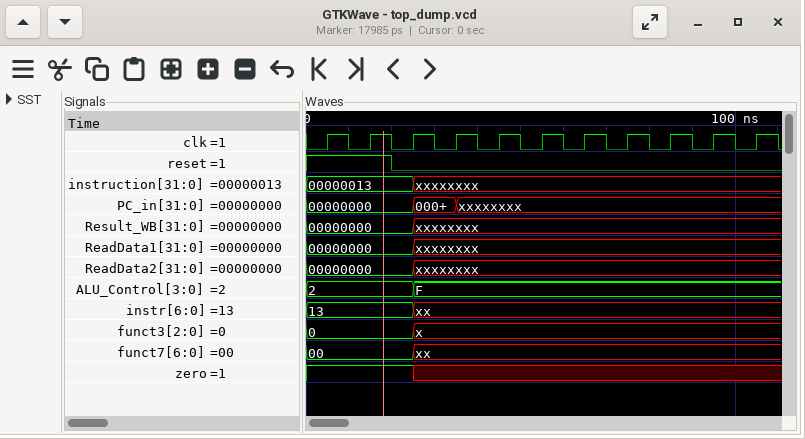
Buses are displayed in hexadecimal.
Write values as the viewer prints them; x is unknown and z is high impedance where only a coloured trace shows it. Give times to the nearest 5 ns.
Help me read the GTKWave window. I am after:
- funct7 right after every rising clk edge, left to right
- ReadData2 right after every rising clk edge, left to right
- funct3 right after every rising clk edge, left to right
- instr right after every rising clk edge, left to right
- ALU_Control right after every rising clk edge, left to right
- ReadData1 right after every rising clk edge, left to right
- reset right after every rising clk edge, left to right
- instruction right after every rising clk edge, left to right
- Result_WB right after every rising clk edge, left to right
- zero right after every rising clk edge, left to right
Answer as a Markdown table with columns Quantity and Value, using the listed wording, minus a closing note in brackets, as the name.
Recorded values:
| Quantity | Value |
|---|---|
| funct7 right after every rising clk edge, left to right | 00, 00, xx, xx, xx, xx, xx, xx, xx, xx, xx |
| ReadData2 right after every rising clk edge, left to right | 00000000, 00000000, xxxxxxxx, xxxxxxxx, xxxxxxxx, xxxxxxxx, xxxxxxxx, xxxxxxxx, xxxxxxxx, xxxxxxxx, xxxxxxxx |
| funct3 right after every rising clk edge, left to right | 0, 0, x, x, x, x, x, x, x, x, x |
| instr right after every rising clk edge, left to right | 13, 13, xx, xx, xx, xx, xx, xx, xx, xx, xx |
| ALU_Control right after every rising clk edge, left to right | 2, 2, F, F, F, F, F, F, F, F, F |
| ReadData1 right after every rising clk edge, left to right | 00000000, 00000000, xxxxxxxx, xxxxxxxx, xxxxxxxx, xxxxxxxx, xxxxxxxx, xxxxxxxx, xxxxxxxx, xxxxxxxx, xxxxxxxx |
| reset right after every rising clk edge, left to right | 1 1 0 0 0 0 0 0 0 0 0 |
| instruction right after every rising clk edge, left to right | 00000013, 00000013, xxxxxxxx, xxxxxxxx, xxxxxxxx, xxxxxxxx, xxxxxxxx, xxxxxxxx, xxxxxxxx, xxxxxxxx, xxxxxxxx |
| Result_WB right after every rising clk edge, left to right | 00000000, 00000000, xxxxxxxx, xxxxxxxx, xxxxxxxx, xxxxxxxx, xxxxxxxx, xxxxxxxx, xxxxxxxx, xxxxxxxx, xxxxxxxx |
| zero right after every rising clk edge, left to right | 1 1 x x x x x x x x x |
